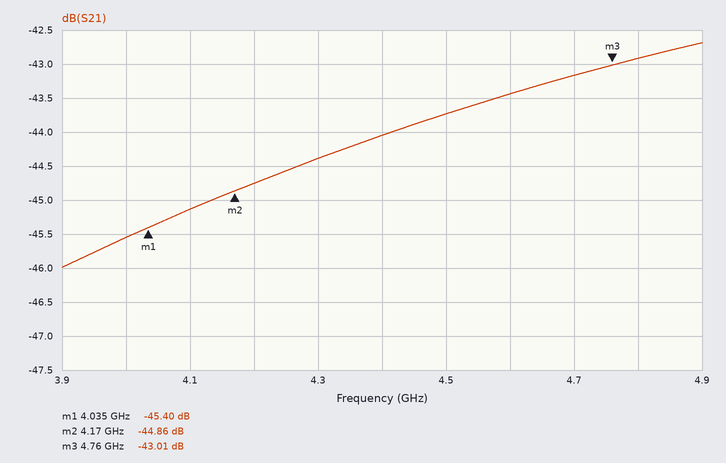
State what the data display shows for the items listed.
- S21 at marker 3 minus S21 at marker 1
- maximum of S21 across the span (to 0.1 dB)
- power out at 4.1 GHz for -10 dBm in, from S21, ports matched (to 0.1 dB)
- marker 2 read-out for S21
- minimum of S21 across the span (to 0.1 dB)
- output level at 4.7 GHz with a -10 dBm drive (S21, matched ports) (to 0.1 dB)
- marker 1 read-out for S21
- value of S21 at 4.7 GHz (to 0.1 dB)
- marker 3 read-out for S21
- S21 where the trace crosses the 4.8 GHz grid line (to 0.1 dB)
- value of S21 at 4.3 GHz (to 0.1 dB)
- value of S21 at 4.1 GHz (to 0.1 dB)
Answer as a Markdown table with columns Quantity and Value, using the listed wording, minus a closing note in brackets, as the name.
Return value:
| Quantity | Value |
|---|---|
| S21 at marker 3 minus S21 at marker 1 | 2.39 dB |
| maximum of S21 across the span | -42.7 dB |
| power out at 4.1 GHz for -10 dBm in, from S21, ports matched | -55.1 dBm |
| marker 2 read-out for S21 | -44.86 dB |
| minimum of S21 across the span | -46.0 dB |
| output level at 4.7 GHz with a -10 dBm drive (S21, matched ports) | -53.2 dBm |
| marker 1 read-out for S21 | -45.40 dB |
| value of S21 at 4.7 GHz | -43.2 dB |
| marker 3 read-out for S21 | -43.01 dB |
| S21 where the trace crosses the 4.8 GHz grid line | -42.9 dB |
| value of S21 at 4.3 GHz | -44.4 dB |
| value of S21 at 4.1 GHz | -45.1 dB |
